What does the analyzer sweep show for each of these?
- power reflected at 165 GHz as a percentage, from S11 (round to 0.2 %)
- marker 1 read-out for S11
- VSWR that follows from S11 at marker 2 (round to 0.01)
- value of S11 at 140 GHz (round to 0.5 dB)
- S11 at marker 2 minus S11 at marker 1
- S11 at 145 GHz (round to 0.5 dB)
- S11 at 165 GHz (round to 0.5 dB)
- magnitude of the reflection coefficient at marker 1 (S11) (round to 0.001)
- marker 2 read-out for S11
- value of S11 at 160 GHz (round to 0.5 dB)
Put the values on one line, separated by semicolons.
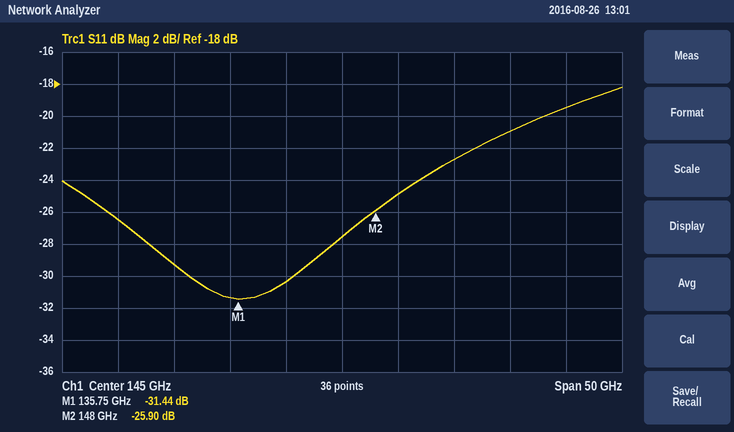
1.2 %; -31.44 dB; 1.11; -30.5 dB; 5.54 dB; -27.5 dB; -19.5 dB; 0.027; -25.90 dB; -21.0 dB
